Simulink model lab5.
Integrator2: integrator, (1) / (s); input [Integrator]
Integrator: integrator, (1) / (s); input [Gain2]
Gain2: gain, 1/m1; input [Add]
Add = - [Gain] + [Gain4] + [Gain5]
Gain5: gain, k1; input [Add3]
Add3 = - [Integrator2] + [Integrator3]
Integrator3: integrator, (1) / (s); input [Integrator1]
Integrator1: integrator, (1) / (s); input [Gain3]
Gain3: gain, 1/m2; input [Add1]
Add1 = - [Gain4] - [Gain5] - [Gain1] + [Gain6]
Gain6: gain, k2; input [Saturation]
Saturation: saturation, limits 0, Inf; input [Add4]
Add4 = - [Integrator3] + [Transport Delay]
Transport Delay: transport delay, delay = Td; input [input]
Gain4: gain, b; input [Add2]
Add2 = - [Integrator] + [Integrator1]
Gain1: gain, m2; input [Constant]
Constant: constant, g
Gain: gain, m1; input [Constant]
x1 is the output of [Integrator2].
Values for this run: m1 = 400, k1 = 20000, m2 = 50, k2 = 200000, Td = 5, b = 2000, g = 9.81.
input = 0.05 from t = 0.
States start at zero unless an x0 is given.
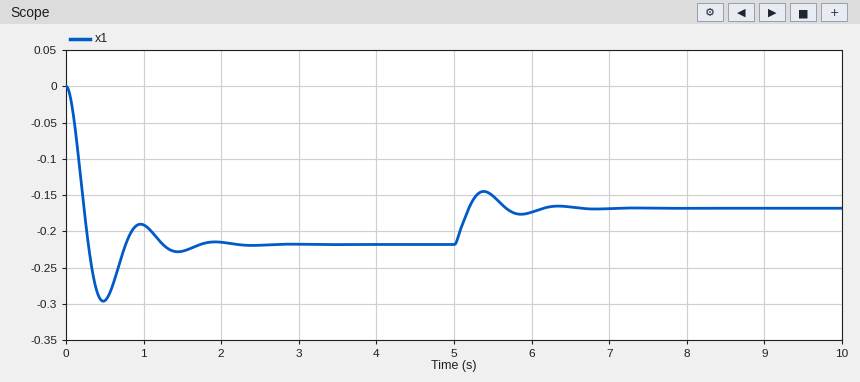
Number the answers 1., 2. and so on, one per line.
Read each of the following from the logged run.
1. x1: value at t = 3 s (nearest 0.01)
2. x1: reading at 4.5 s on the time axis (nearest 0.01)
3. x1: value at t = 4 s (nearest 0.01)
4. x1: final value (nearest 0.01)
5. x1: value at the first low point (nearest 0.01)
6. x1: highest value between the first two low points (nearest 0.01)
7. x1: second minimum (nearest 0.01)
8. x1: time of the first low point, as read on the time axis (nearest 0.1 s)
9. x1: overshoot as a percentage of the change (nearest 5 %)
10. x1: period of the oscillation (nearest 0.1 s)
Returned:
1. -0.22
2. -0.22
3. -0.22
4. -0.17
5. -0.30
6. -0.19
7. -0.23
8. 0.5 s
9. 75 %
10. 1.0 s
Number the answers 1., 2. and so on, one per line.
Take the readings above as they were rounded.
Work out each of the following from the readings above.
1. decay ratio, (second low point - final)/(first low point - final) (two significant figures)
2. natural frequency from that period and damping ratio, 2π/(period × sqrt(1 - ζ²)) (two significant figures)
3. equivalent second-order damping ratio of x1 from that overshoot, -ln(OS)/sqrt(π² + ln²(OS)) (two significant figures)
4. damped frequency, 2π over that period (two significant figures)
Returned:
1. 0.46
2. 6.3 rad/s
3. 0.091
4. 6.3 rad/s
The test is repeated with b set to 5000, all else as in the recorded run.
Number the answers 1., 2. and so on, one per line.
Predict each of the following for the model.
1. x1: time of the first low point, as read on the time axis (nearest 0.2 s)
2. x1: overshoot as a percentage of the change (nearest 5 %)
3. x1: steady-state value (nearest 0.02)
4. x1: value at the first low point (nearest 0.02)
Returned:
1. 0.8 s
2. 30 %
3. -0.16
4. -0.22
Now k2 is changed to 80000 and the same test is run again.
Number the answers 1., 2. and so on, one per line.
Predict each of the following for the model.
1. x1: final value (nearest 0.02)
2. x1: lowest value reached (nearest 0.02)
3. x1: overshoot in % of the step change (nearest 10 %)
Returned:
1. -0.20
2. -0.36
3. 80 %
